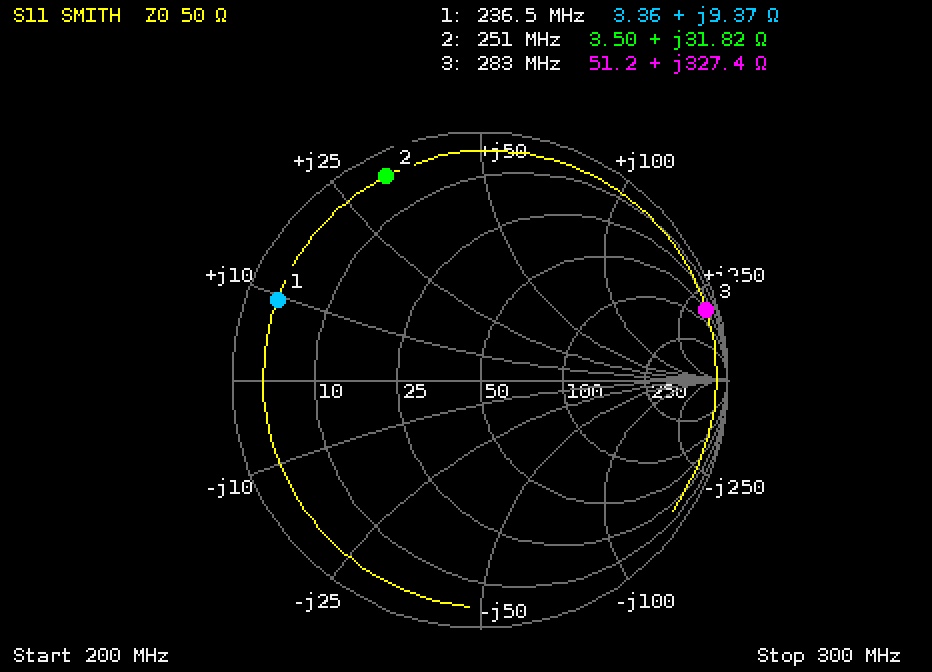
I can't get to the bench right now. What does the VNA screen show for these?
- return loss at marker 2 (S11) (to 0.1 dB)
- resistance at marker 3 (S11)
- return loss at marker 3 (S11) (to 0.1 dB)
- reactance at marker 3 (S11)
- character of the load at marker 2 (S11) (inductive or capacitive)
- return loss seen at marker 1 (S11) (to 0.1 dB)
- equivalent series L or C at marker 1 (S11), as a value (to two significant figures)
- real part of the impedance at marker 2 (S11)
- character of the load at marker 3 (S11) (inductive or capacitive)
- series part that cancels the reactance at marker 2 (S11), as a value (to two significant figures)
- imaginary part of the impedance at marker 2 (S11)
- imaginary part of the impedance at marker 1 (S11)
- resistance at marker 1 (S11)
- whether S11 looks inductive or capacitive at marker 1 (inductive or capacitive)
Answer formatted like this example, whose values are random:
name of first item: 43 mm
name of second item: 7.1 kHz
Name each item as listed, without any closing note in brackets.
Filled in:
return loss at marker 2 (S11): 0.9 dB
resistance at marker 3: 51.2 Ω
return loss at marker 3 (S11): 0.4 dB
reactance at marker 3: +327.4 Ω
character of the load at marker 2 (S11): inductive
return loss seen at marker 1 (S11): 1.1 dB
equivalent series L or C at marker 1 (S11), as a value: 6.3 nH
real part of the impedance at marker 2: 3.50 Ω
character of the load at marker 3 (S11): inductive
series part that cancels the reactance at marker 2 (S11), as a value: 20 pF
imaginary part of the impedance at marker 2: +31.82 Ω
imaginary part of the impedance at marker 1: +9.37 Ω
resistance at marker 1: 3.36 Ω
whether S11 looks inductive or capacitive at marker 1: inductive
